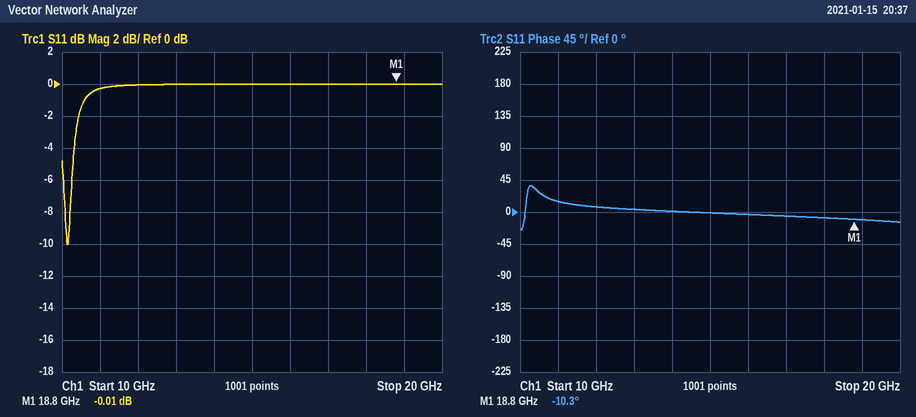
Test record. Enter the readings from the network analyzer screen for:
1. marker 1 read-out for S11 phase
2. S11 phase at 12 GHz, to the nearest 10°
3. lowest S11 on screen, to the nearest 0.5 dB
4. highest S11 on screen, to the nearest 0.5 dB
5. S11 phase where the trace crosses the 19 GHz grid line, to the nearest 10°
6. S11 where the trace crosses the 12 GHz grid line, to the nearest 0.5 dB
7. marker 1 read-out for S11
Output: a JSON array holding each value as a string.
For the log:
["-10.3°", "10°", "-10.0 dB", "0.0 dB", "-10°", "0.0 dB", "-0.01 dB"]
